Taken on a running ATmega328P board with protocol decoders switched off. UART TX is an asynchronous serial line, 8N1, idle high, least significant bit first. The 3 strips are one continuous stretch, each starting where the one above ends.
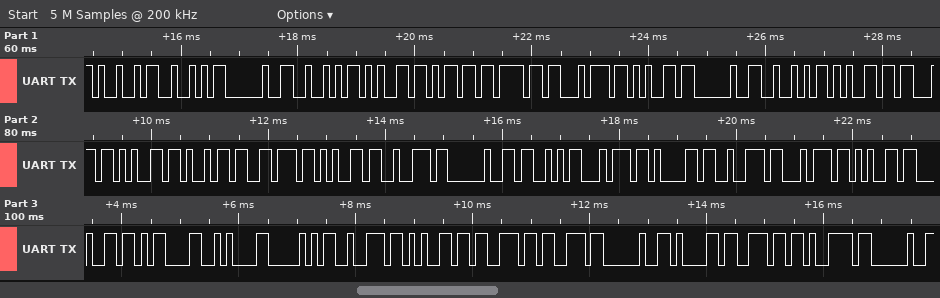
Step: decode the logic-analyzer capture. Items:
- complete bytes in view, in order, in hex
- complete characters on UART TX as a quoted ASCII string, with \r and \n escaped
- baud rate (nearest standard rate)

49 52 20 52 65 6D 6F 74 65 20 52 65 63 65 69 76 65 72 20 53 74 61 72 74 65 64 0D 0A 50 72 65 73 73 20 61 6E 79 20
"IR Remote Receiver Started\r\nPress any "
9600 baud
